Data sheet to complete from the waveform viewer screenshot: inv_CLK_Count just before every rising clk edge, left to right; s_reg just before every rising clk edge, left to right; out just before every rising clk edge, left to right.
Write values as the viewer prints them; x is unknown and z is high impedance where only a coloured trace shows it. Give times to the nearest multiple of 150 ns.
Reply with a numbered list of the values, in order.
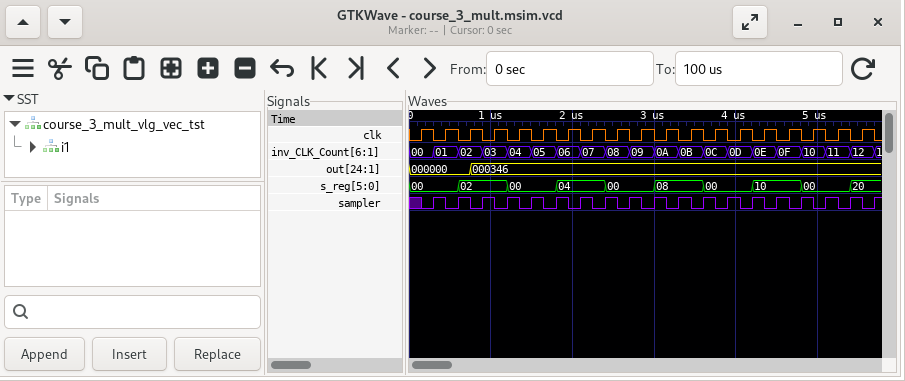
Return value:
1. 00, 01, 02, 03, 04, 05, 06, 07, 08, 09, 0A, 0B, 0C, 0D, 0E, 0F, 10, 11, 12
2. 00, 00, 02, 02, 00, 00, 04, 04, 00, 00, 08, 08, 00, 00, 10, 10, 00, 00, 20
3. 000000, 000000, 000000, 000346, 000346, 000346, 000346, 000346, 000346, 000346, 000346, 000346, 000346, 000346, 000346, 000346, 000346, 000346, 000346
